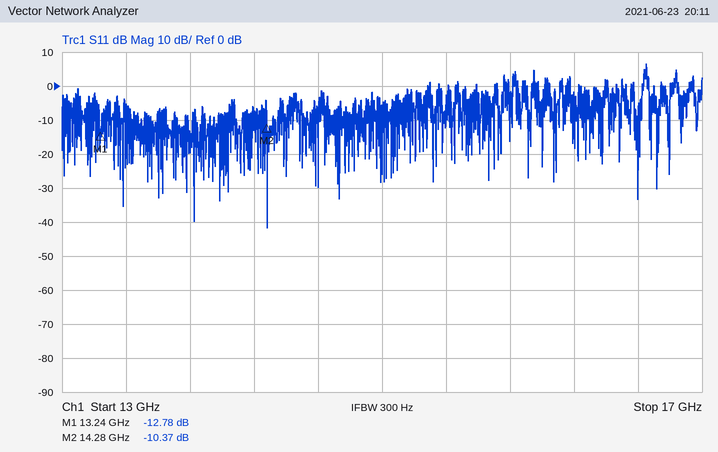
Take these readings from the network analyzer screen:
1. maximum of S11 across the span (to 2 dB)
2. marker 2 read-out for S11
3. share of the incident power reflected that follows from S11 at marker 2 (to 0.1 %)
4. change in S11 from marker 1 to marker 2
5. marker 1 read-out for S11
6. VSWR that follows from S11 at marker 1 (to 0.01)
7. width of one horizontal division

6 dB
-10.37 dB
9.2 %
2.41 dB
-12.78 dB
1.60
400 MHz
